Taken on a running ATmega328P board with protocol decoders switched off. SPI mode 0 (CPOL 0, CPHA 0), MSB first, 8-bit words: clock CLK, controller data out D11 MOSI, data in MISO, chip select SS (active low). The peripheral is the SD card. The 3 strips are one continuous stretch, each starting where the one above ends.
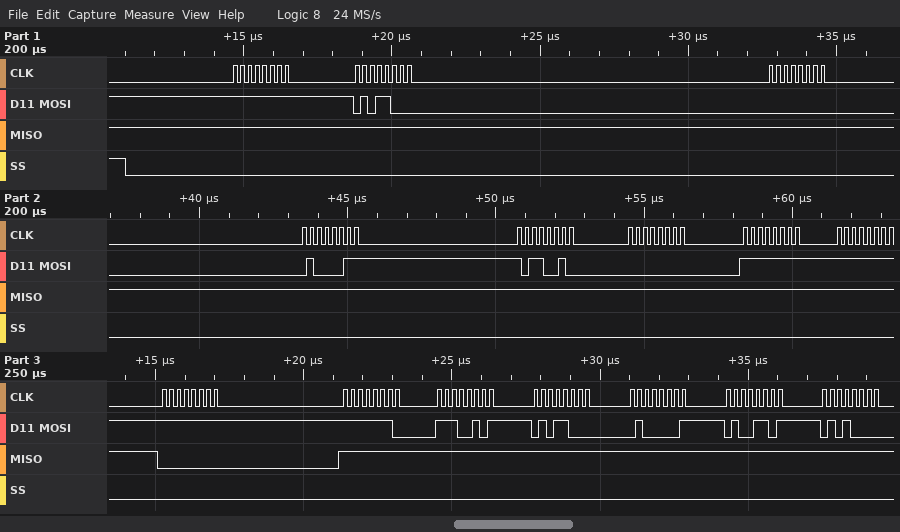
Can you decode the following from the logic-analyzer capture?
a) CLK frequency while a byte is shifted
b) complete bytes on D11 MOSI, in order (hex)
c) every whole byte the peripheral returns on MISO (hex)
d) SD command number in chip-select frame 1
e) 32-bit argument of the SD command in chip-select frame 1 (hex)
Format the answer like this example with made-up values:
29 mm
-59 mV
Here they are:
4 MHz
FF 58 00 43 B2 00 FF FF FF FE E5 58 41 4D 50
FF FF FF FF FF FF FF FF 00 FF FF FF FF FF FF
CMD24
0x0043B200
